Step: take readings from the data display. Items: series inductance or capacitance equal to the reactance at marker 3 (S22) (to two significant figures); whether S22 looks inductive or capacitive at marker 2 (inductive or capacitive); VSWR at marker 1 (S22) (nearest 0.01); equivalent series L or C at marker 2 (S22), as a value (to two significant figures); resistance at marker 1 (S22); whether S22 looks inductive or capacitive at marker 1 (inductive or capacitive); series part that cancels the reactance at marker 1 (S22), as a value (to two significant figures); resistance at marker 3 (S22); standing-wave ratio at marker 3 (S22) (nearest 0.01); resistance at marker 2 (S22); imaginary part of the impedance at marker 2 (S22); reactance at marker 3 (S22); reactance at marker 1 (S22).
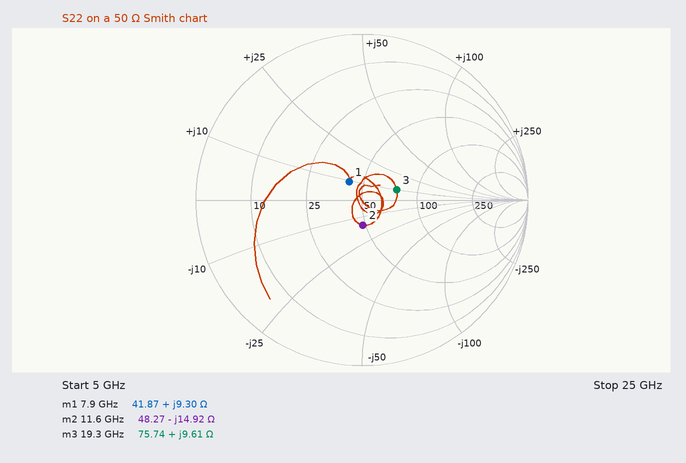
79 pH
capacitive
1.31
920 fF
41.87 Ω
inductive
2.2 pF
75.74 Ω
1.56
48.27 Ω
-14.92 Ω
+9.61 Ω
+9.30 Ω
